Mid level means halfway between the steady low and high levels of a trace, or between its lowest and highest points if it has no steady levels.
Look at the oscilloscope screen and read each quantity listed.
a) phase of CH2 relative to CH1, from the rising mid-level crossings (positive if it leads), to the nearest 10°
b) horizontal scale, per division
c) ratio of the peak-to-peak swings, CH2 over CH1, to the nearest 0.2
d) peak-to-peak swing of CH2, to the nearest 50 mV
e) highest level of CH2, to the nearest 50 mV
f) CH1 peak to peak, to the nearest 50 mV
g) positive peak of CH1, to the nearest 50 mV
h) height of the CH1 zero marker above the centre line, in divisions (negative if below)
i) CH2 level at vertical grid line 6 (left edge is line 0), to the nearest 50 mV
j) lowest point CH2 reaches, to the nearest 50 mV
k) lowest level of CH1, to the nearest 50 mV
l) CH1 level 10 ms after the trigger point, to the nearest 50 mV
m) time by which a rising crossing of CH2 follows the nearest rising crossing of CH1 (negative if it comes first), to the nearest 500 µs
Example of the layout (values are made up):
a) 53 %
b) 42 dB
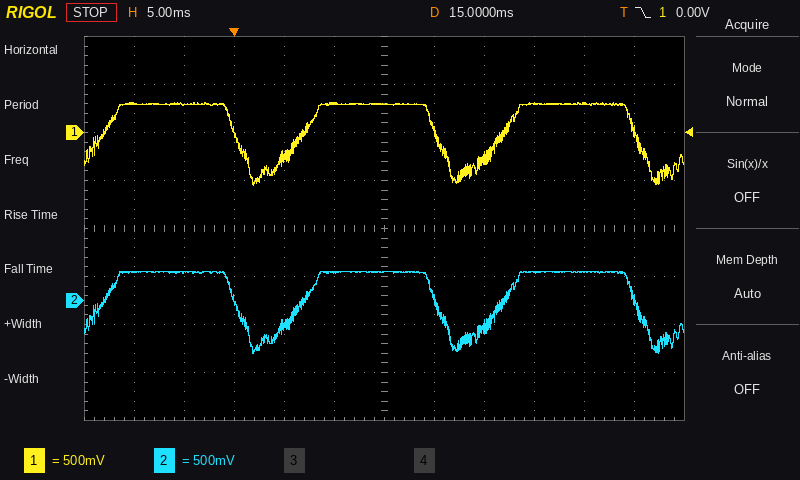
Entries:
a) 0°
b) 5 ms
c) 1.0
d) 850 mV
e) 300 mV
f) 850 mV
g) 300 mV
h) +2.0 div
i) 300 mV
j) -550 mV
k) -550 mV
l) 300 mV
m) 0.0 ms
